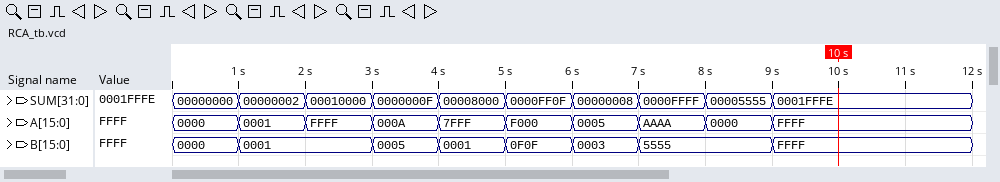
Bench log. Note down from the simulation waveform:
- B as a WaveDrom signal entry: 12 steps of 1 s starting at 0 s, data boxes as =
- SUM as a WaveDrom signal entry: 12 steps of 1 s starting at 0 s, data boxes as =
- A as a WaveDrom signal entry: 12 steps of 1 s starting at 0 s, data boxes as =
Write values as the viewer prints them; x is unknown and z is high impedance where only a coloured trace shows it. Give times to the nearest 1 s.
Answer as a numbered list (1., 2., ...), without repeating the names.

1. {name: 'B', wave: '==.=====.=..', data: '0000 0001 0005 0001 0F0F 0003 5555 FFFF'}
2. {name: 'SUM', wave: '==========..', data: '00000000 00000002 00010000 0000000F 00008000 0000FF0F 00000008 0000FFFF 00005555 0001FFFE'}
3. {name: 'A', wave: '==========..', data: '0000 0001 FFFF 000A 7FFF F000 0005 AAAA 0000 FFFF'}
